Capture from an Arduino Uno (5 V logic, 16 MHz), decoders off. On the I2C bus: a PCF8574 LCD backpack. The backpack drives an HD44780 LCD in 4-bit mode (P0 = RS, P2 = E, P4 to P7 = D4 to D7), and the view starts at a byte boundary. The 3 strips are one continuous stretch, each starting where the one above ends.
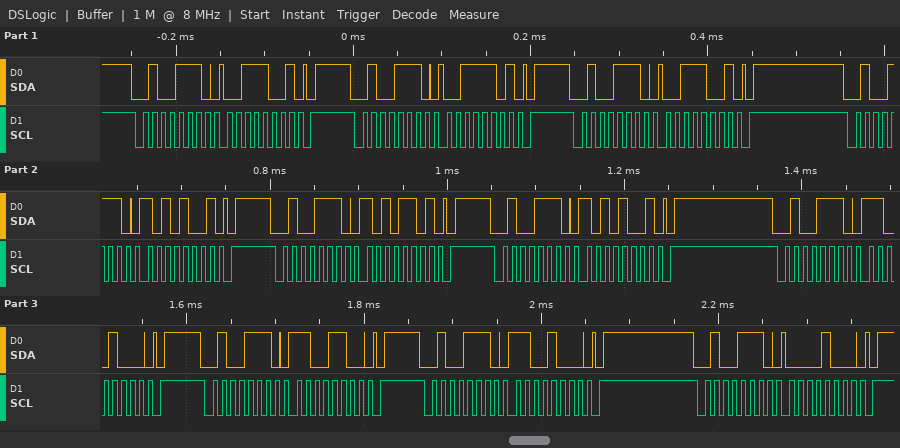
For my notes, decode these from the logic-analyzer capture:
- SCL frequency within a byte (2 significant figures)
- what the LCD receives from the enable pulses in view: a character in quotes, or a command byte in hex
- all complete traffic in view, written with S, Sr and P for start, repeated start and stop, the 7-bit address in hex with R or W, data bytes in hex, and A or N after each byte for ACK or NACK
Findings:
100 kHz
':'
S 27W A 39 A P S 27W A 3D A P S 27W A 39 A P S 27W A A9 A P S 27W A AD A P S 27W A A9 A P S 27W A C8 A P S 27W A CC A P S 27W A C8 A P S 27W A 08 A P
